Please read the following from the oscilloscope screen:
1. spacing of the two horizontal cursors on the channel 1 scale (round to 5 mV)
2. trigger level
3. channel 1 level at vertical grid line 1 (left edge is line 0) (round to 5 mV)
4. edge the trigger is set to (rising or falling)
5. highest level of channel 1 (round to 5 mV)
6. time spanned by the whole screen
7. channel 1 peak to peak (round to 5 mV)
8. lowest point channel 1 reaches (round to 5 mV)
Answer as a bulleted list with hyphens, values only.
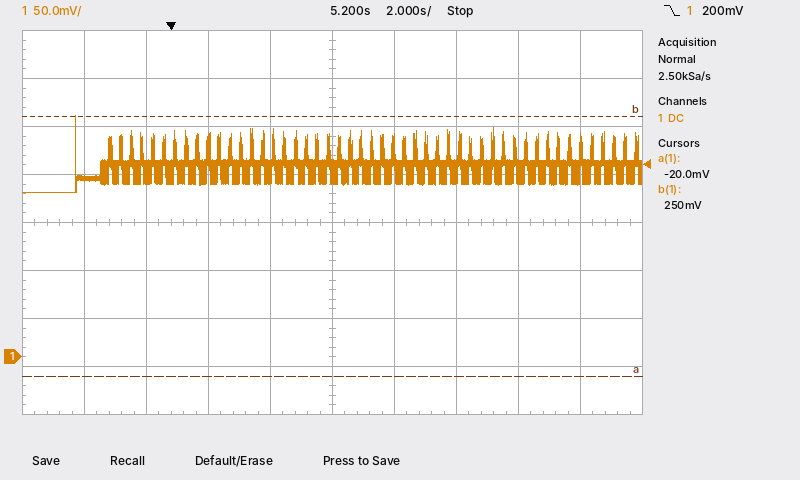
- 270 mV
- 200 mV
- 185 mV
- falling
- 250 mV
- 20 s
- 80 mV
- 170 mV
